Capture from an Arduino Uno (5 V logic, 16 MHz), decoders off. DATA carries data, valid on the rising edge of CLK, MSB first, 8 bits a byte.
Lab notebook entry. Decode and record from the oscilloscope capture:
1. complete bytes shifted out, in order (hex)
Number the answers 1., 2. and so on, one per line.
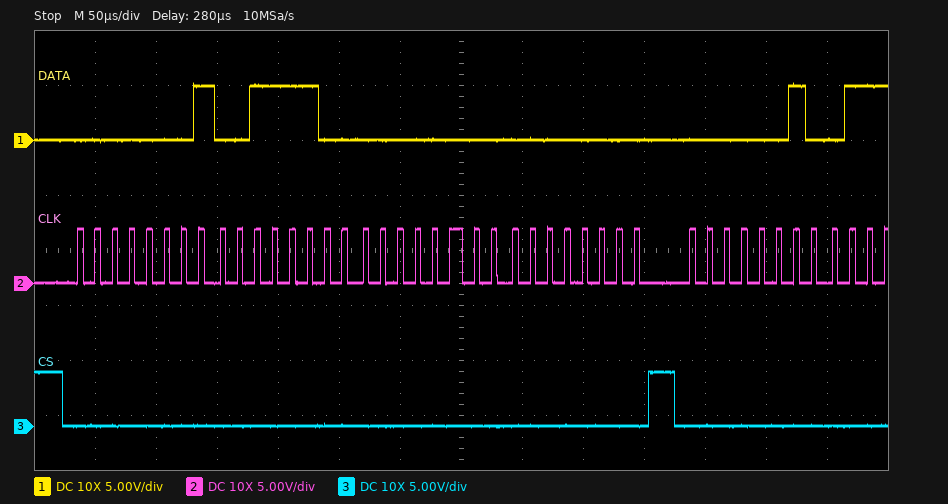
1. 01 3C 00 00 02
